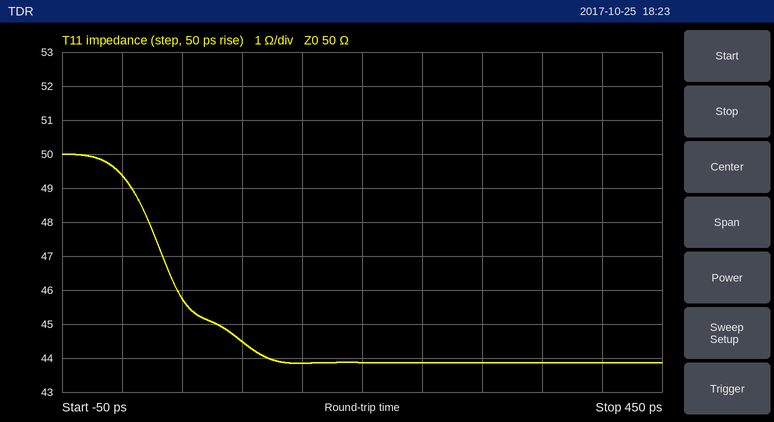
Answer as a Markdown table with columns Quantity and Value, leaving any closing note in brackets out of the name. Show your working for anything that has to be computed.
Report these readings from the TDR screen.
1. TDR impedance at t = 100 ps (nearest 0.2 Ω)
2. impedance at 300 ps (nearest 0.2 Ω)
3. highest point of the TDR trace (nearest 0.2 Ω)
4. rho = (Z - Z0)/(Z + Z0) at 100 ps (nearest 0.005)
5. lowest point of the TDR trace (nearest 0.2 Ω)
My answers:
| Quantity | Value |
|---|---|
| TDR impedance at t = 100 ps | 44.4 Ω |
| impedance at 300 ps | 43.8 Ω |
| highest point of the TDR trace | 50.0 Ω |
| rho = (Z - Z0)/(Z + Z0) at 100 ps | (44.4 − 50)/(44.4 + 50) ≈ -0.0593, so -0.060 to the nearest 0.005 |
| lowest point of the TDR trace | 43.8 Ω |
